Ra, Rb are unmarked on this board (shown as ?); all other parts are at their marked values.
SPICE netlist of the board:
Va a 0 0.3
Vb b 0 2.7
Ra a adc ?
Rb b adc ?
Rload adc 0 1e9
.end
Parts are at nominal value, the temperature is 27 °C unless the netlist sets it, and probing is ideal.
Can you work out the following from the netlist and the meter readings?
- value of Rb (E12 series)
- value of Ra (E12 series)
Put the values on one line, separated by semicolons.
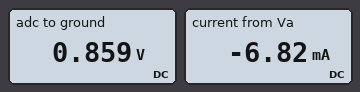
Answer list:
270 Ω; 82 Ω
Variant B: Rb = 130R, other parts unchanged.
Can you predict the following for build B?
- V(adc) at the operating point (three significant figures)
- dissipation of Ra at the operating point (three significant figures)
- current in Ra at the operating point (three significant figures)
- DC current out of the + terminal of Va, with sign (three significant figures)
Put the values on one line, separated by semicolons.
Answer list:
1.23 V; 10.5 mW; 11.3 mA; -11.3 mA
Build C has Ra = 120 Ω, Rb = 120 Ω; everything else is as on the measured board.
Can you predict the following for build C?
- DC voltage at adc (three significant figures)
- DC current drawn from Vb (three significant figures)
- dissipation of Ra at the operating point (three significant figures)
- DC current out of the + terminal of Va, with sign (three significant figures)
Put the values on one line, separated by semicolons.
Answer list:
1.50 V; 10.0 mA; 12.0 mW; -10.0 mA
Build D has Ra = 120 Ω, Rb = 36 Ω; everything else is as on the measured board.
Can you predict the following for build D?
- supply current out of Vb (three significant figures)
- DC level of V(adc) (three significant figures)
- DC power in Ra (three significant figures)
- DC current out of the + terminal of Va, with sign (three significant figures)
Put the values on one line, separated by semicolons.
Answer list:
15.4 mA; 2.15 V; 28.4 mW; -15.4 mA
